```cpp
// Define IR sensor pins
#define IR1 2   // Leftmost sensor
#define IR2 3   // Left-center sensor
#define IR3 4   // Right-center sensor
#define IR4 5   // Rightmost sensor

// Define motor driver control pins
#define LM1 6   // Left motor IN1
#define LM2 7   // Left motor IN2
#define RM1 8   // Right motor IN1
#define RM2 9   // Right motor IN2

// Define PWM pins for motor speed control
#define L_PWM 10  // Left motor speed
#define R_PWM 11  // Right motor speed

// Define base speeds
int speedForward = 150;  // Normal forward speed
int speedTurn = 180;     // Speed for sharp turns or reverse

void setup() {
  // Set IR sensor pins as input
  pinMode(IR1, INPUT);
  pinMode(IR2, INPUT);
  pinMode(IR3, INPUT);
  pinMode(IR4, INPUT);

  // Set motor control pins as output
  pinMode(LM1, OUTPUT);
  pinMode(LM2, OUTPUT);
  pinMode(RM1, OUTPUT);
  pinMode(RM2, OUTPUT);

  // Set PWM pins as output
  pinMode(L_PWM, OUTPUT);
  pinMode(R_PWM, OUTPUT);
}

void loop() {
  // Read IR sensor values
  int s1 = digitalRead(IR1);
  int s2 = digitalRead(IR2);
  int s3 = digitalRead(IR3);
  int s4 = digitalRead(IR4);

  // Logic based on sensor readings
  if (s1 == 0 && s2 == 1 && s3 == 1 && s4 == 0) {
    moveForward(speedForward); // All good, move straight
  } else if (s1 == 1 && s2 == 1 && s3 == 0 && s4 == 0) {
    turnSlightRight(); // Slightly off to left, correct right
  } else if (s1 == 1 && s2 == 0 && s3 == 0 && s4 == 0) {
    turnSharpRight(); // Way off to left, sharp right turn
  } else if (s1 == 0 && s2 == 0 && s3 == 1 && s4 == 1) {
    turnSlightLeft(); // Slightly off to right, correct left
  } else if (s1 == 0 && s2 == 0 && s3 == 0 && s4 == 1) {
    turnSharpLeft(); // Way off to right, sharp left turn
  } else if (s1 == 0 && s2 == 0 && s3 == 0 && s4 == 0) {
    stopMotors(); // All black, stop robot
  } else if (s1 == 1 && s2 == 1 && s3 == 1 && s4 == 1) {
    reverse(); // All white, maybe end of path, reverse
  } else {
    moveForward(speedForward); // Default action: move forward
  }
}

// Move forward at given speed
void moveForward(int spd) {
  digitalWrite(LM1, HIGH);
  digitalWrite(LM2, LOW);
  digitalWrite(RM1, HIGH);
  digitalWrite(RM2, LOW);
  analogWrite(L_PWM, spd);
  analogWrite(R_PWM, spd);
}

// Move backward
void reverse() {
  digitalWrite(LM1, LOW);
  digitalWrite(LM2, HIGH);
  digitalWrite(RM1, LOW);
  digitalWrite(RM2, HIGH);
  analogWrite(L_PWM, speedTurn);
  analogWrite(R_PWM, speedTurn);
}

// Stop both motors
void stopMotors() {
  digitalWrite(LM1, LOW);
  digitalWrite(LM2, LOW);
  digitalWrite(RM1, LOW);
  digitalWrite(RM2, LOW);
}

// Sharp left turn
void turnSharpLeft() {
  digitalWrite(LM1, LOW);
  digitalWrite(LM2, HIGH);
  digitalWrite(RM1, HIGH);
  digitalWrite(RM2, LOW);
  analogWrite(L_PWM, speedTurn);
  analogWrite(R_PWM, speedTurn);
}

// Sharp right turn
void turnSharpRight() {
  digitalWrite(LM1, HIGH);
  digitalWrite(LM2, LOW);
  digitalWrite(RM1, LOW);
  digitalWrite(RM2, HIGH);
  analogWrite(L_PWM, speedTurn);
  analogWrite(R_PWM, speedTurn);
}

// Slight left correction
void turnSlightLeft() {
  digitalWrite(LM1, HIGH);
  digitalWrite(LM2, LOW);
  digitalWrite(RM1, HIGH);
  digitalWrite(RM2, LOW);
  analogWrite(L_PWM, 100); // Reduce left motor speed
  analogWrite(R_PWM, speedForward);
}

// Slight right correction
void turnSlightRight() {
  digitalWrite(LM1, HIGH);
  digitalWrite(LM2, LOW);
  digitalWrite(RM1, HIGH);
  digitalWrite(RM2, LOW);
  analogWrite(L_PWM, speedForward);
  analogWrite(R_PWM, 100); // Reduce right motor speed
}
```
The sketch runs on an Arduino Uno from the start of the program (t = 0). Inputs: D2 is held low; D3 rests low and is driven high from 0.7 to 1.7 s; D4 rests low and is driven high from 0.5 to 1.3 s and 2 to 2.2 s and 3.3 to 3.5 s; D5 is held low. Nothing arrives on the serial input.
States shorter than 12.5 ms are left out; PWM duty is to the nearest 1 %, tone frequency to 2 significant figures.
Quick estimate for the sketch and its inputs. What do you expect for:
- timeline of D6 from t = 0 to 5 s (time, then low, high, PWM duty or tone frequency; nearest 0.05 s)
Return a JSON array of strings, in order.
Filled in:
["0 s low; 0.5 s high; 1.7 s low; 2 s high; 2.2 s low; 3.3 s high; 3.5 s low"]
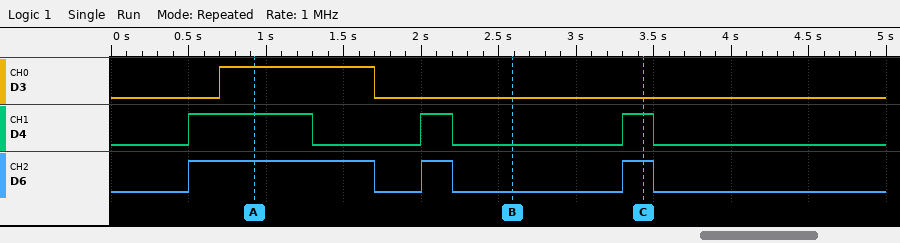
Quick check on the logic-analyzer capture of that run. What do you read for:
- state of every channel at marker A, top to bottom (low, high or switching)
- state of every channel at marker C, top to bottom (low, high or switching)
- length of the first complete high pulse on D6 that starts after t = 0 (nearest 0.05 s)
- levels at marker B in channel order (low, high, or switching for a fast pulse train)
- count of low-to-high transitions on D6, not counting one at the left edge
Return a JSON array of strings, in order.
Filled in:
["D3 high, D4 high, D6 high", "D3 low, D4 high, D6 high", "1.20 s", "D3 low, D4 low, D6 low", "3"]
